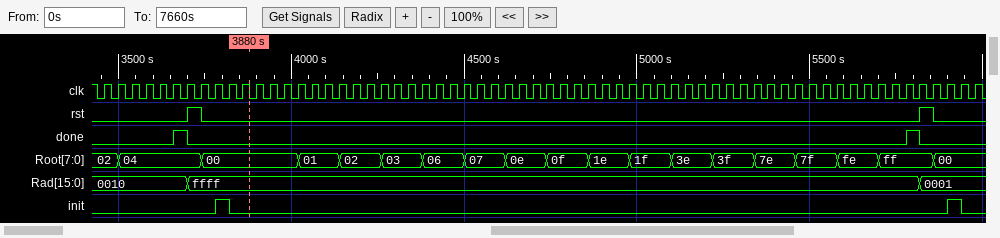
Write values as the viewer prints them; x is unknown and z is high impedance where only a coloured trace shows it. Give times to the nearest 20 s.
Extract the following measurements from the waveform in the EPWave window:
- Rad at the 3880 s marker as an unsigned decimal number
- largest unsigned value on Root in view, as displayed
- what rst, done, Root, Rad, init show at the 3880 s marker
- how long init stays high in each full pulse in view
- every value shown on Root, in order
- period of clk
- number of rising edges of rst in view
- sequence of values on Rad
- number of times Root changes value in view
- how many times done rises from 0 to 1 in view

65535
ff
rst=0, done=0, Root=00, Rad=ffff, init=0
40 s, 40 s
02, 04, 00, 01, 02, 03, 06, 07, 0e, 0f, 1e, 1f, 3e, 3f, 7e, 7f, fe, ff, 00
40 s
2
0010, ffff, 0001
18
2
